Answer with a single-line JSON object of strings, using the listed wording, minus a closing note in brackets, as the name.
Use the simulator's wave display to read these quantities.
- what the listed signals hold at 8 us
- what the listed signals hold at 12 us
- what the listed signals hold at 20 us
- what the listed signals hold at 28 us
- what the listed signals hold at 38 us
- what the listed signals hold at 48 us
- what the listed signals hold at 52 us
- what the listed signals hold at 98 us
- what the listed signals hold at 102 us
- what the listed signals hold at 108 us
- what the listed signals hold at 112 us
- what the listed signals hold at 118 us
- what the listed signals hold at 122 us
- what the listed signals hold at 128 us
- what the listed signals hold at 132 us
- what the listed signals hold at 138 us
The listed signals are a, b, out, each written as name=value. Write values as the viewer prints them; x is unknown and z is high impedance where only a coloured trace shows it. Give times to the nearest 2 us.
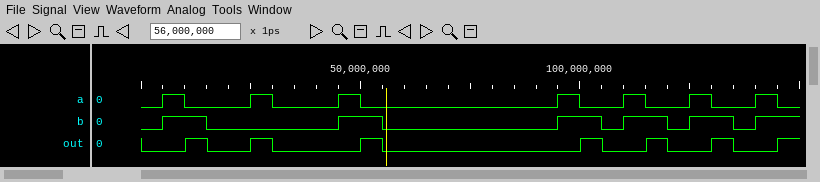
{"what the listed signals hold at 8 us": "a=1, b=1, out=0", "what the listed signals hold at 12 us": "a=0, b=1, out=1", "what the listed signals hold at 20 us": "a=0, b=0, out=0", "what the listed signals hold at 28 us": "a=1, b=0, out=1", "what the listed signals hold at 38 us": "a=0, b=0, out=0", "what the listed signals hold at 48 us": "a=1, b=1, out=0", "what the listed signals hold at 52 us": "a=0, b=1, out=1", "what the listed signals hold at 98 us": "a=1, b=1, out=0", "what the listed signals hold at 102 us": "a=0, b=1, out=1", "what the listed signals hold at 108 us": "a=0, b=0, out=0", "what the listed signals hold at 112 us": "a=1, b=1, out=0", "what the listed signals hold at 118 us": "a=0, b=1, out=1", "what the listed signals hold at 122 us": "a=0, b=0, out=0", "what the listed signals hold at 128 us": "a=1, b=1, out=0", "what the listed signals hold at 132 us": "a=0, b=1, out=1", "what the listed signals hold at 138 us": "a=0, b=0, out=0"}
